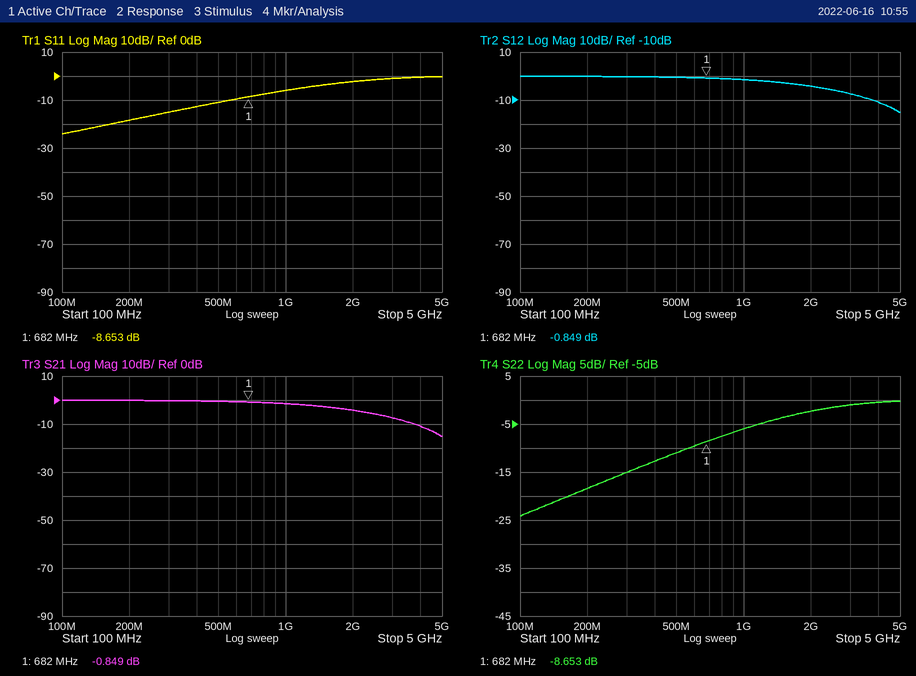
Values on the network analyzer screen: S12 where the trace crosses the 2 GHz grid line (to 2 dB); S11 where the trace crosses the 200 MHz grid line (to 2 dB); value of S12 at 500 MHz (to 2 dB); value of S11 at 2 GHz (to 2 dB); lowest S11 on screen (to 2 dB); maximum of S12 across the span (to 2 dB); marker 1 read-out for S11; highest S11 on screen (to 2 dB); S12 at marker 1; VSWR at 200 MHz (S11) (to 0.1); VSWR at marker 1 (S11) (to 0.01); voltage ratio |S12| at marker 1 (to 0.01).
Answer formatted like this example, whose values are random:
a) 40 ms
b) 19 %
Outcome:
a) -4 dB
b) -18 dB
c) 0 dB
d) -2 dB
e) -24 dB
f) 0 dB
g) -8.653 dB
h) 0 dB
i) -0.849 dB
j) 1.3
k) 2.17
l) 0.91
